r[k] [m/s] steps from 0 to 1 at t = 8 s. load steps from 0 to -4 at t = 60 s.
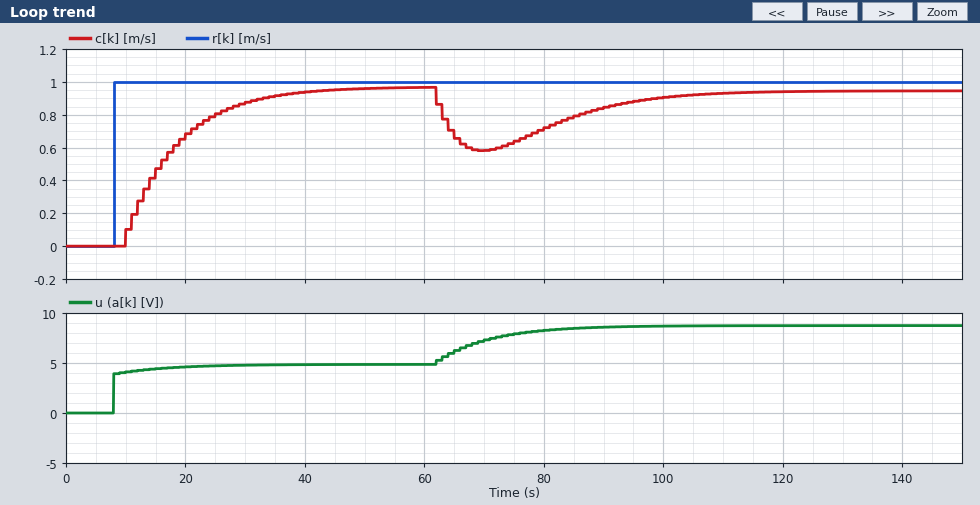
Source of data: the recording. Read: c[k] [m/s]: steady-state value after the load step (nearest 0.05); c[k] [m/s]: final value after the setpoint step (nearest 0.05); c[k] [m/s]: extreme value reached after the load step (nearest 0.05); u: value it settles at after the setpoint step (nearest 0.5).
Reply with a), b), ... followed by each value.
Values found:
a) 0.95
b) 0.95
c) 0.60
d) 5.0
